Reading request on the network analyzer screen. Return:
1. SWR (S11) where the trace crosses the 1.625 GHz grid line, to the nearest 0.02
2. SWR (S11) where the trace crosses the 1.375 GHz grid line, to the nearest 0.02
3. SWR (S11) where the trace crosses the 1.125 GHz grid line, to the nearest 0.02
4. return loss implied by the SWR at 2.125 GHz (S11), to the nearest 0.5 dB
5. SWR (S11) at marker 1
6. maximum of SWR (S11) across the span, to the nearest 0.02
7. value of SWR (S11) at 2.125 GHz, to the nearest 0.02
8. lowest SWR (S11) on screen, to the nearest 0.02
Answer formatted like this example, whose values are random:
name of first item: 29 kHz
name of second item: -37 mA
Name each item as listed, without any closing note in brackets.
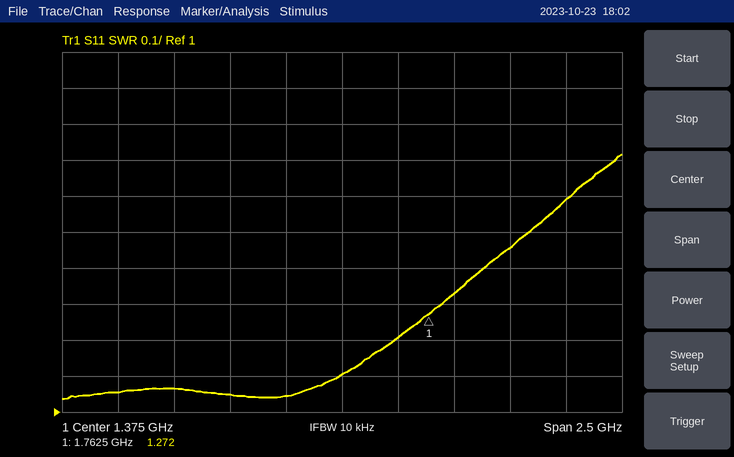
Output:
SWR (S11) where the trace crosses the 1.625 GHz grid line, to the nearest 0.02: 1.20
SWR (S11) where the trace crosses the 1.375 GHz grid line, to the nearest 0.02: 1.10
SWR (S11) where the trace crosses the 1.125 GHz grid line, to the nearest 0.02: 1.04
return loss implied by the SWR at 2.125 GHz (S11), to the nearest 0.5 dB: 14.5 dB
SWR (S11) at marker 1: 1.272
maximum of SWR (S11) across the span, to the nearest 0.02: 1.72
value of SWR (S11) at 2.125 GHz, to the nearest 0.02: 1.46
lowest SWR (S11) on screen, to the nearest 0.02: 1.04
